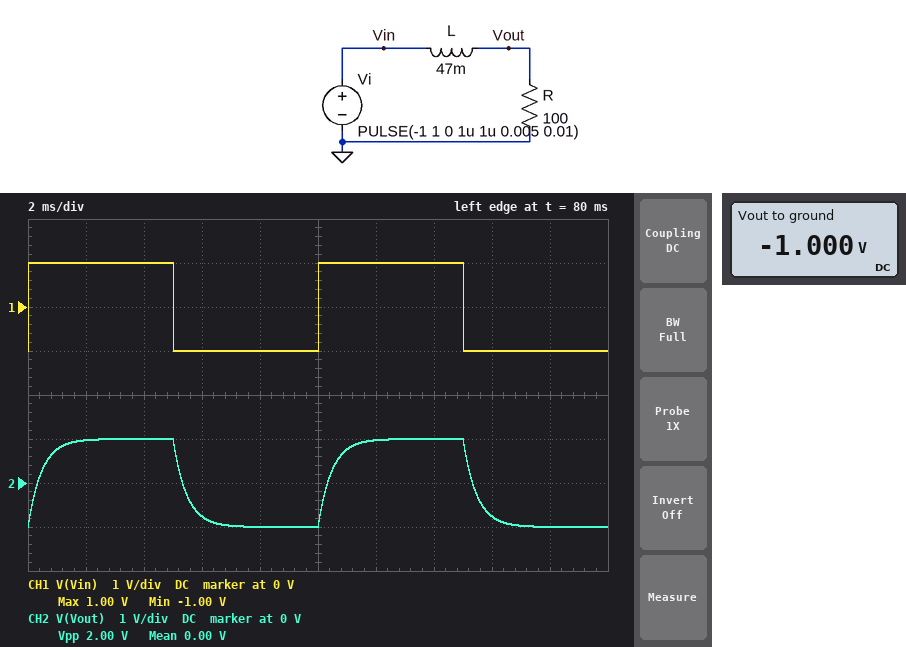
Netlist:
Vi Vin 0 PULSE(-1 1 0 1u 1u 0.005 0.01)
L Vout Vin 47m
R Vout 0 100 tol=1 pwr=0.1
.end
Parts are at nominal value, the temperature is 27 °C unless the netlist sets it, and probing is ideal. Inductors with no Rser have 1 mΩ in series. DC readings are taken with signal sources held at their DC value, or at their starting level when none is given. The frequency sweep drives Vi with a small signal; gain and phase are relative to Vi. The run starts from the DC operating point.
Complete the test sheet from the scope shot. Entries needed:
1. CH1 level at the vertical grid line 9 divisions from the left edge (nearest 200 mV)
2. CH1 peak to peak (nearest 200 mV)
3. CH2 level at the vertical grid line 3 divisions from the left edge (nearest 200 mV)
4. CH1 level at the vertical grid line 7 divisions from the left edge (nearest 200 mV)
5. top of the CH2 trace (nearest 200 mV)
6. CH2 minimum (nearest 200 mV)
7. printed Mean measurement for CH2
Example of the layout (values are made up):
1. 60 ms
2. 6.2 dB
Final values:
1. -1.0 V
2. 2.0 V
3. -800 mV
4. 1.0 V
5. 1.0 V
6. -1.0 V
7. 0.00 V
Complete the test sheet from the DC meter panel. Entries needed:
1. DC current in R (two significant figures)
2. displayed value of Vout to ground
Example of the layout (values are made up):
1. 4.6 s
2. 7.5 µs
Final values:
1. 10 mA
2. -1.000 V
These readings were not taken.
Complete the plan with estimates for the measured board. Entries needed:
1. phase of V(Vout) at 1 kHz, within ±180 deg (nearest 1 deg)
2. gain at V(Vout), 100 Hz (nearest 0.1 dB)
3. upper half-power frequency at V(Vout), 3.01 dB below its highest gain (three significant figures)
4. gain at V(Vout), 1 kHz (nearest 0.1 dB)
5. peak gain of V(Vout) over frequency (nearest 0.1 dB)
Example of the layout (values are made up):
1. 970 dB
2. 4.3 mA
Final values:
1. -71 deg
2. -0.4 dB
3. 339 Hz
4. -9.9 dB
5. 0 dB
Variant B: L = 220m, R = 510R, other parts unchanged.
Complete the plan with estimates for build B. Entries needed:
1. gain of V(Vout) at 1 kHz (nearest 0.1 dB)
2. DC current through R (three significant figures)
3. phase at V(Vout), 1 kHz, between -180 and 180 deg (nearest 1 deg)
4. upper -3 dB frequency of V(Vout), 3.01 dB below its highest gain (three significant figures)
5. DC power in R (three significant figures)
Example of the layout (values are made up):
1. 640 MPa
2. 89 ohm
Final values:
1. -9.2 dB
2. 1.96 mA
3. -70 deg
4. 369 Hz
5. 1.96 mW
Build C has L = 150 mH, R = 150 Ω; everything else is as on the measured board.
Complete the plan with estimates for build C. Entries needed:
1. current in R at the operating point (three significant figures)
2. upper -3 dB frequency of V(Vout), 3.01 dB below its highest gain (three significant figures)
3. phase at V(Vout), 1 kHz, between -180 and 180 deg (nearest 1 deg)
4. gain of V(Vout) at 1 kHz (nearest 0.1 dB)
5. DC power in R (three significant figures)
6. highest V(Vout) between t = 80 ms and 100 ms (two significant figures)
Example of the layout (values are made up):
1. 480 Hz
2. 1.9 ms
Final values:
1. 6.67 mA
2. 159 Hz
3. -81 deg
4. -16.1 dB
5. 6.67 mW
6. 990 mV
